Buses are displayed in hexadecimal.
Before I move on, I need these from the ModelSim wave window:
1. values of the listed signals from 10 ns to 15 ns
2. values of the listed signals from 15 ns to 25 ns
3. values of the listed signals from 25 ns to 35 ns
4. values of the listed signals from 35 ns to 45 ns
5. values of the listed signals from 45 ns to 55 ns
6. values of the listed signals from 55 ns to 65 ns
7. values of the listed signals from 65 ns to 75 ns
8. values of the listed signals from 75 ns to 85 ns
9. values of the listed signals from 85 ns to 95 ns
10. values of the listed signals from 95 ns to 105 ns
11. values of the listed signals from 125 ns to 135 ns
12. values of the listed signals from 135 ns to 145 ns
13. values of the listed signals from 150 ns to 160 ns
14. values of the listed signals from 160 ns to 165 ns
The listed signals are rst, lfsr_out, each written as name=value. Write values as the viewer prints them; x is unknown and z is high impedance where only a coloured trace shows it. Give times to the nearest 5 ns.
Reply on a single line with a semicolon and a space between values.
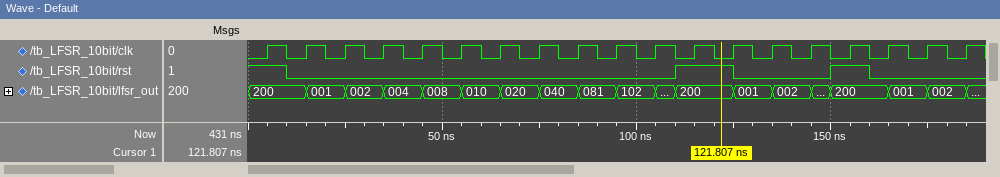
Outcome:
rst=0, lfsr_out=200; rst=0, lfsr_out=001; rst=0, lfsr_out=002; rst=0, lfsr_out=004; rst=0, lfsr_out=008; rst=0, lfsr_out=010; rst=0, lfsr_out=020; rst=0, lfsr_out=040; rst=0, lfsr_out=081; rst=0, lfsr_out=102; rst=0, lfsr_out=001; rst=0, lfsr_out=002; rst=1, lfsr_out=200; rst=0, lfsr_out=200
